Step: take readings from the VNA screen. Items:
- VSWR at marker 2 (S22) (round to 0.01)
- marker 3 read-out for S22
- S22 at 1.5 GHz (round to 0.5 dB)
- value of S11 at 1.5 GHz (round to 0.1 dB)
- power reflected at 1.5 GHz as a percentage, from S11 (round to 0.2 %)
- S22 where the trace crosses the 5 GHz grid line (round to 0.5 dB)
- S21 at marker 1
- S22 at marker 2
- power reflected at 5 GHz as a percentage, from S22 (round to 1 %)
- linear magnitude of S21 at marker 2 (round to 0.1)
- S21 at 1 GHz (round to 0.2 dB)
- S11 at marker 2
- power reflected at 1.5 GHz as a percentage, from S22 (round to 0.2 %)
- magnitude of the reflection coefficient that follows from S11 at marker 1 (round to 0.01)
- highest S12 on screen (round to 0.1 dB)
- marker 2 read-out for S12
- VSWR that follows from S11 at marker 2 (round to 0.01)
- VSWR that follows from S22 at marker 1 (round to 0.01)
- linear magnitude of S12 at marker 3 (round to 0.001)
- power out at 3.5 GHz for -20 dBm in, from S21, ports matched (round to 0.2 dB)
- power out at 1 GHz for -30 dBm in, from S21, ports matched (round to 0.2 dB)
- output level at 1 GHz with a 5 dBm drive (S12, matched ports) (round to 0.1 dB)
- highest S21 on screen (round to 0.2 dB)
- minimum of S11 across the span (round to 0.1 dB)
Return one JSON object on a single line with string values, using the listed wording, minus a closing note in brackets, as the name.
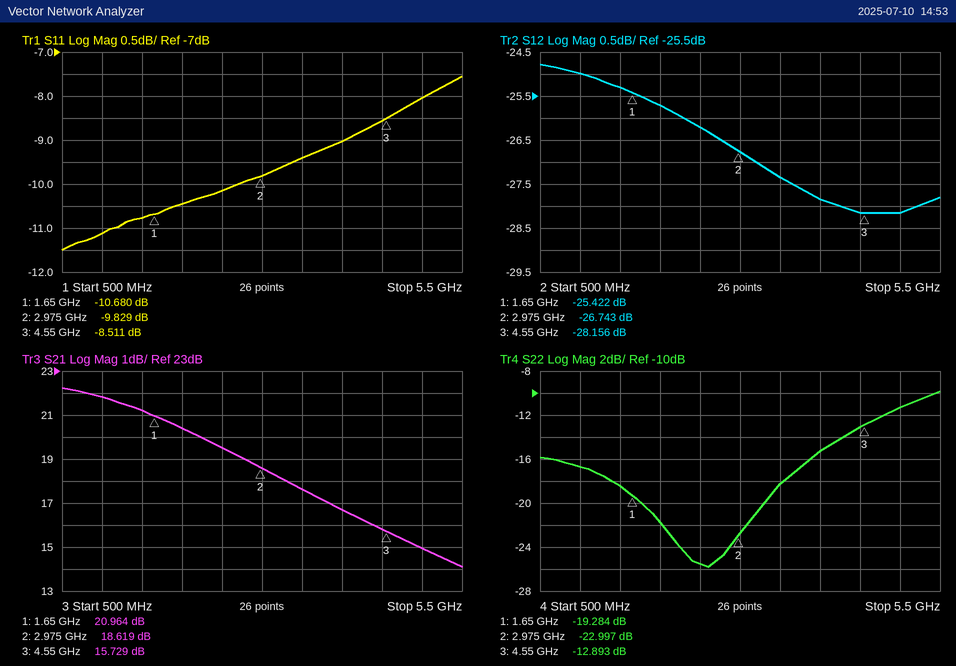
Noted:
{"VSWR at marker 2 (S22)": "1.15", "marker 3 read-out for S22": "-12.893 dB", "S22 at 1.5 GHz": "-18.5 dB", "value of S11 at 1.5 GHz": "-10.8 dB", "power reflected at 1.5 GHz as a percentage, from S11": "8.4 %", "S22 where the trace crosses the 5 GHz grid line": "-11.5 dB", "S21 at marker 1": "20.964 dB", "S22 at marker 2": "-22.997 dB", "power reflected at 5 GHz as a percentage, from S22": "7 %", "linear magnitude of S21 at marker 2": "8.5", "S21 at 1 GHz": "21.8 dB", "S11 at marker 2": "-9.829 dB", "power reflected at 1.5 GHz as a percentage, from S22": "1.4 %", "magnitude of the reflection coefficient that follows from S11 at marker 1": "0.29", "highest S12 on screen": "-24.8 dB", "marker 2 read-out for S12": "-26.743 dB", "VSWR that follows from S11 at marker 2": "1.95", "VSWR that follows from S22 at marker 1": "1.24", "linear magnitude of S12 at marker 3": "0.039", "power out at 3.5 GHz for -20 dBm in, from S21, ports matched": "-2.4 dBm", "power out at 1 GHz for -30 dBm in, from S21, ports matched": "-8.2 dBm", "output level at 1 GHz with a 5 dBm drive (S12, matched ports)": "-20.0 dBm", "highest S21 on screen": "22.2 dB", "minimum of S11 across the span": "-11.5 dB"}
